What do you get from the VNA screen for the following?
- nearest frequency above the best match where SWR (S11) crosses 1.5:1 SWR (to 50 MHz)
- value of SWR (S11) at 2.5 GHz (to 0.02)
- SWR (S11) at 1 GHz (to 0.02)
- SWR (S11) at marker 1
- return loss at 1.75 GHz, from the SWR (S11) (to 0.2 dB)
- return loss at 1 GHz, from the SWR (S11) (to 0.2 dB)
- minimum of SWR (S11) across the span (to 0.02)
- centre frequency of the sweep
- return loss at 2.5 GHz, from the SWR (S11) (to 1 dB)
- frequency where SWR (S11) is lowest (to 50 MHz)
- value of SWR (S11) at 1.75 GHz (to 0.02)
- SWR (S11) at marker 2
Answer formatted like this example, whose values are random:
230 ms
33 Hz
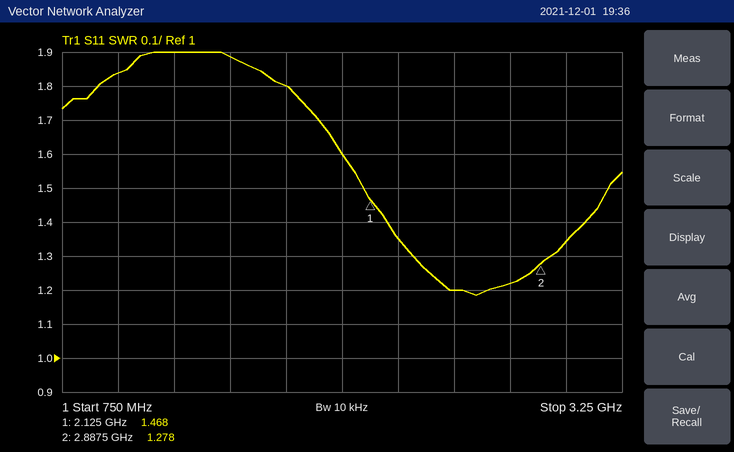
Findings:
3.20 GHz
1.20
1.84
1.468
10.8 dB
10.6 dB
1.18
2 GHz
21 dB
2.60 GHz
1.80
1.278
